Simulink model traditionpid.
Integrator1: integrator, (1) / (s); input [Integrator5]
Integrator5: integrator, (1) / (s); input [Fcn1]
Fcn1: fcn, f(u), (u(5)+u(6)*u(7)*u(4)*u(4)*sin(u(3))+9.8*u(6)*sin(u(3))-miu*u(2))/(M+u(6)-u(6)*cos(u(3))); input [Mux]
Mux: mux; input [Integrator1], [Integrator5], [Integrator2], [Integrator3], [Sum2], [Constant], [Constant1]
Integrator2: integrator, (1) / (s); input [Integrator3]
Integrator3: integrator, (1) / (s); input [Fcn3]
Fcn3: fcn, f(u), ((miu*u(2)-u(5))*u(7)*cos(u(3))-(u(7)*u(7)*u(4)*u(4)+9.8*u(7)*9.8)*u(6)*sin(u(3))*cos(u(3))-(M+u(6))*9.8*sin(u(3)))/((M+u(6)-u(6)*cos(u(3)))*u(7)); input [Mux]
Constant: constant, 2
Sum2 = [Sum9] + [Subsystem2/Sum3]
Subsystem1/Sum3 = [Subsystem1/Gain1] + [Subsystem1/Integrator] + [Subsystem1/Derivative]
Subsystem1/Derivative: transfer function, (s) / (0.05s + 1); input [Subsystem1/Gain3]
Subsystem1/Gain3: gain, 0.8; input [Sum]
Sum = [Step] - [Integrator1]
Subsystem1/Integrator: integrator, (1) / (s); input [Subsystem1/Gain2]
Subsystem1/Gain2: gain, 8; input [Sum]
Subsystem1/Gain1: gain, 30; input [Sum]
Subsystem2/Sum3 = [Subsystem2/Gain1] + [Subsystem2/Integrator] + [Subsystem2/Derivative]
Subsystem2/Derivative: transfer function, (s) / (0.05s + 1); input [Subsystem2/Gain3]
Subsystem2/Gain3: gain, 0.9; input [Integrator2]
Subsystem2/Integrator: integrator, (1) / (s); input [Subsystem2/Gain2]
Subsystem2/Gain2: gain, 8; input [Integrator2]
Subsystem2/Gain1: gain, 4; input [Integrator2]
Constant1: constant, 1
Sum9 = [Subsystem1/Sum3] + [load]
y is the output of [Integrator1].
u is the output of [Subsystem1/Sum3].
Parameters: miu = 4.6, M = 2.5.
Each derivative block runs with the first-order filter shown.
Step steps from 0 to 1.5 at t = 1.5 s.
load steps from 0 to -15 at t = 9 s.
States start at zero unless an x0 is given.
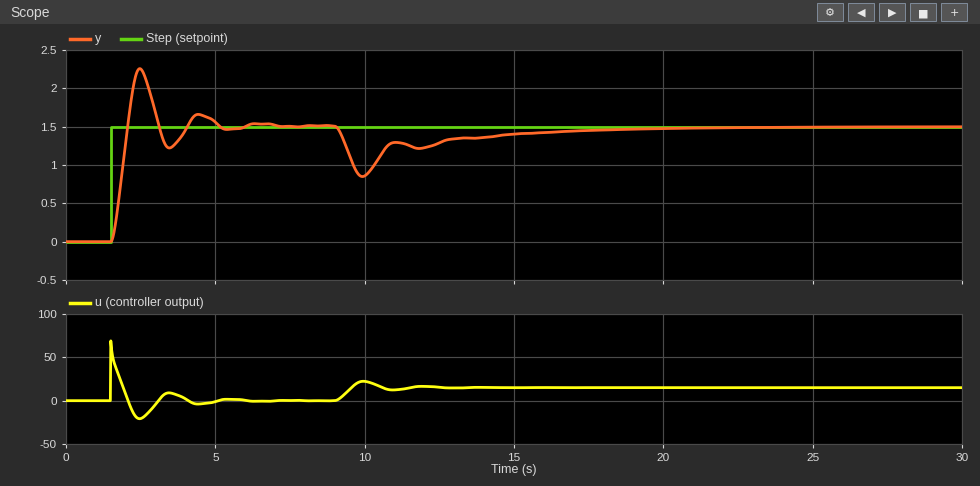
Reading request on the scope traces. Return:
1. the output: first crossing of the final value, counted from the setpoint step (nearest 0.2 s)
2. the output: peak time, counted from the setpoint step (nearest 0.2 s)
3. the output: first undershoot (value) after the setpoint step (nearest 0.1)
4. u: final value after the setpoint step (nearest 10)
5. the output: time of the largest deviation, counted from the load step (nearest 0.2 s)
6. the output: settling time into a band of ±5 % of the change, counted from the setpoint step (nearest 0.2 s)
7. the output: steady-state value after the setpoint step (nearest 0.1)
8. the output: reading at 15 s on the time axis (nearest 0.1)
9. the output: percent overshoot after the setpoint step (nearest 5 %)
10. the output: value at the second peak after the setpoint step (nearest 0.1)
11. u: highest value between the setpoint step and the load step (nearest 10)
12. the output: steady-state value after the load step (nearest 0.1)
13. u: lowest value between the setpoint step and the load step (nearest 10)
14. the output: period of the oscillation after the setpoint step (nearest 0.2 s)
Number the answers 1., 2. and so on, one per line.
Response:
1. 0.6 s
2. 1.0 s
3. 1.2
4. 0
5. 1.0 s
6. 3.4 s
7. 1.5
8. 1.4
9. 50 %
10. 1.7
11. 70
12. 1.5
13. -20
14. 2.0 s
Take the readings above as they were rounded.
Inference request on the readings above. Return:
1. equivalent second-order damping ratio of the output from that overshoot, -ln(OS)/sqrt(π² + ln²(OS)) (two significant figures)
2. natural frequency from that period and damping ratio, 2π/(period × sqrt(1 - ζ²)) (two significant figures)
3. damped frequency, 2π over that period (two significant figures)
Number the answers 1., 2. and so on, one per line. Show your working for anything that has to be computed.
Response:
1. ln(0.5) = -0.693; 0.693 / sqrt(9.870 + 0.480) = 0.22
2. 2π / (2 × sqrt(1 - 0.22²)) = 3.2 rad/s
3. 2π / 2 = 3.1 rad/s
